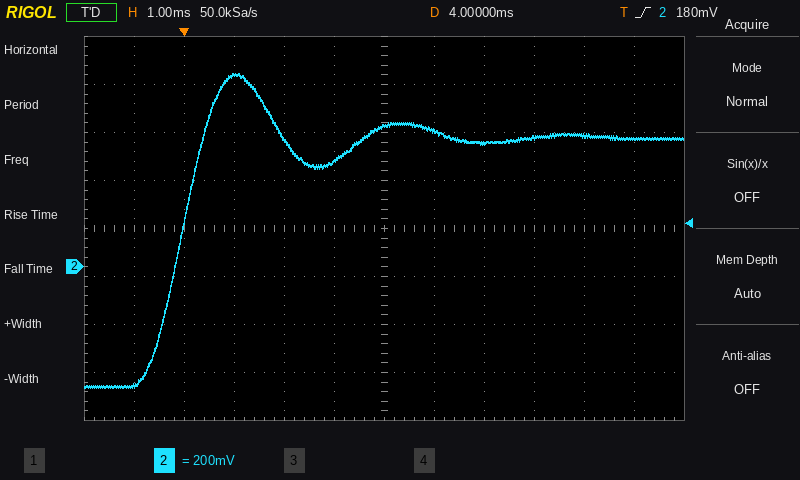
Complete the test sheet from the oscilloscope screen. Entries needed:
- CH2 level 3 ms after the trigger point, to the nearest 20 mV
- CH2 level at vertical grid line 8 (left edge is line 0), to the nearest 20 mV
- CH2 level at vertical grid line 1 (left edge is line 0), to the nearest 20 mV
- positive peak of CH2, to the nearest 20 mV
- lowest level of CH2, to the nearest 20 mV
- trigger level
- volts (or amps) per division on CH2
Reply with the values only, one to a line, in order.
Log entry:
440 mV
520 mV
-500 mV
800 mV
-500 mV
180 mV
200 mV
